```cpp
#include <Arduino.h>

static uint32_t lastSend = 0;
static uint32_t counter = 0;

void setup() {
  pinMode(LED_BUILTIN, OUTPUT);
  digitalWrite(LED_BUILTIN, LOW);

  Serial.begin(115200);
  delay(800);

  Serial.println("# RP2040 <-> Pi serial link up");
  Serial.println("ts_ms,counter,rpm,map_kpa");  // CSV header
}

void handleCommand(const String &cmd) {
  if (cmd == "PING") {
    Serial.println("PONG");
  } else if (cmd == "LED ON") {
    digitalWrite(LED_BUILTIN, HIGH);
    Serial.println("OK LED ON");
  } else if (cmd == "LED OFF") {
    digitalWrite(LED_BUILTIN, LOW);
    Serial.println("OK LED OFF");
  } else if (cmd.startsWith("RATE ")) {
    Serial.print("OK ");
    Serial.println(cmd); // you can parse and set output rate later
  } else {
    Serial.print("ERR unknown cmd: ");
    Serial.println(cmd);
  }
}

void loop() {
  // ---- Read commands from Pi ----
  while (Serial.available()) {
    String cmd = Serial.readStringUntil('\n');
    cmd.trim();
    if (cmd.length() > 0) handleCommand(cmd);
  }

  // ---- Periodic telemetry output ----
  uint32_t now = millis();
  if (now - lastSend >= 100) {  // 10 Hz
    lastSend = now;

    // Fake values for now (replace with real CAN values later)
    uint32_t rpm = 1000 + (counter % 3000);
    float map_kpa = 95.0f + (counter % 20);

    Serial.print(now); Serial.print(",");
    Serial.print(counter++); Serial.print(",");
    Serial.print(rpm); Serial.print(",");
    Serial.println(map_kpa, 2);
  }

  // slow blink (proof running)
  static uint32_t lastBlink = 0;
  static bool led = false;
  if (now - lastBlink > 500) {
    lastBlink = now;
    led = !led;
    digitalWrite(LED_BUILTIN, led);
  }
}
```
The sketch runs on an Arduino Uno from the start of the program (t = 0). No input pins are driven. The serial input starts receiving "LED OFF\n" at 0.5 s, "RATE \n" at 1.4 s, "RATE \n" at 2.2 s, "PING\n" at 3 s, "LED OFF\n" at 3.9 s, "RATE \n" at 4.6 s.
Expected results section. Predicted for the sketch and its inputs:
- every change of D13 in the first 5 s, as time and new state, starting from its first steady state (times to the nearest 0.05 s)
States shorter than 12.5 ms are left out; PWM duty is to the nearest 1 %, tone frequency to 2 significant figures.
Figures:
0 s low; 0.8 s high; 1.3 s low; 1.8 s high; 2.3 s low; 2.8 s high; 3.3 s low; 3.8 s high; 3.9 s low; 4.8 s high
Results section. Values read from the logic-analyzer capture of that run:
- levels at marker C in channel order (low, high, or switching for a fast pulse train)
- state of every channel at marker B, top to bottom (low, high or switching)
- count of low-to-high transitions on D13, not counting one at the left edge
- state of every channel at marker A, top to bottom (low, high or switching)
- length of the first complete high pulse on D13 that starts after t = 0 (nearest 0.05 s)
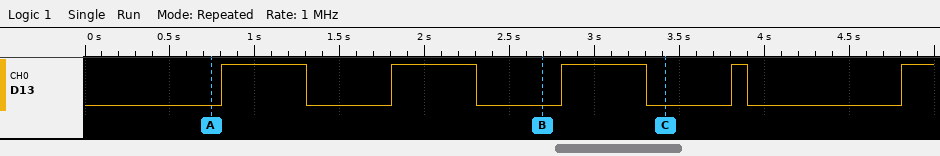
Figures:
D13 low
D13 low
5
D13 low
0.50 s
